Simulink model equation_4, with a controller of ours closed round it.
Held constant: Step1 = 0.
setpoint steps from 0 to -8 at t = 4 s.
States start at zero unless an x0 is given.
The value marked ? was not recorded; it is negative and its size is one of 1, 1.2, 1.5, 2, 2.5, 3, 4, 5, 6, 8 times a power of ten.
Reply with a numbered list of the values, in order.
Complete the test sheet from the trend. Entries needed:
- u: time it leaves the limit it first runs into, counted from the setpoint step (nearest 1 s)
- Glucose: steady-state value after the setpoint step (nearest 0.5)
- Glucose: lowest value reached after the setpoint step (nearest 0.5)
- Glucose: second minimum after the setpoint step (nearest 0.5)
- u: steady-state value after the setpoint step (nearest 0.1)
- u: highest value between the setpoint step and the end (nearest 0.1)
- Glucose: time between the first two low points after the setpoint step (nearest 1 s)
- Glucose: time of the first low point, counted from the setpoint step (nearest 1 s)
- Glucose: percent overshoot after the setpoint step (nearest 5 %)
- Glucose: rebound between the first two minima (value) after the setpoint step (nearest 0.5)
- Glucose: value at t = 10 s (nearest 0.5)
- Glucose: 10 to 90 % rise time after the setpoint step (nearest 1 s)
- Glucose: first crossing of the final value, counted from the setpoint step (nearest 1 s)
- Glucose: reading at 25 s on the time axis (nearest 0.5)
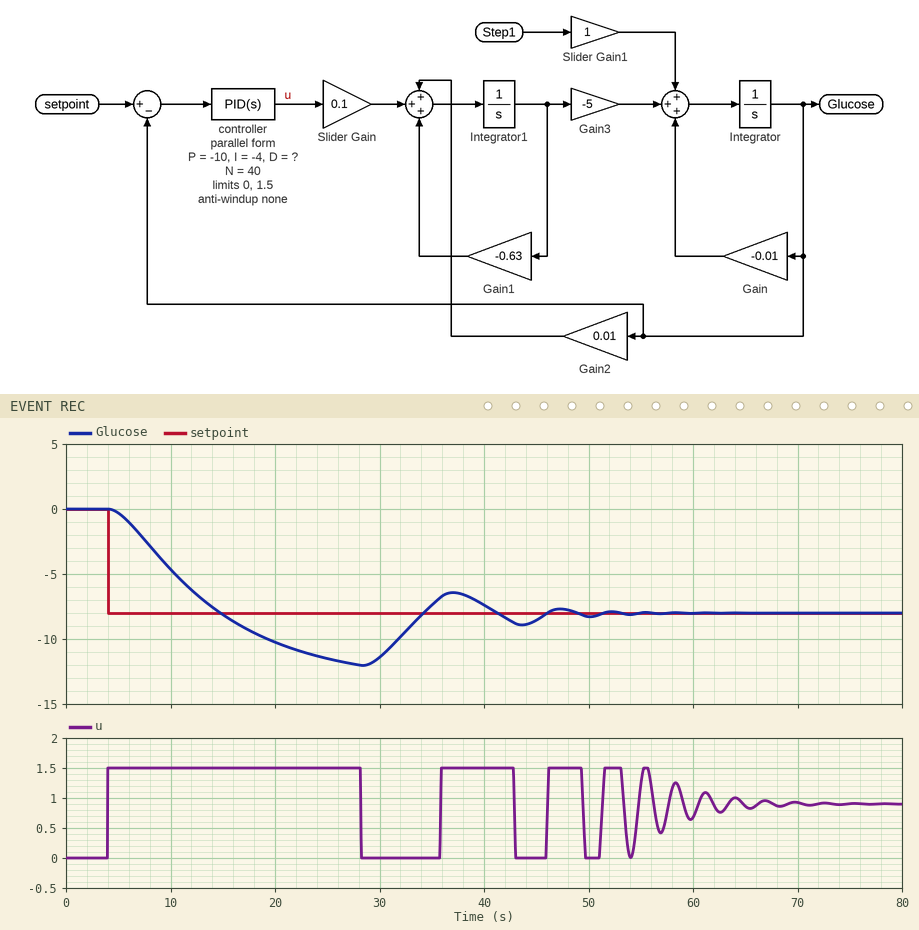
1. 24 s
2. -8.0
3. -12.0
4. -9.0
5. 0.9
6. 1.5
7. 15 s
8. 24 s
9. 50 %
10. -6.5
11. -4.5
12. 8 s
13. 11 s
14. -11.5
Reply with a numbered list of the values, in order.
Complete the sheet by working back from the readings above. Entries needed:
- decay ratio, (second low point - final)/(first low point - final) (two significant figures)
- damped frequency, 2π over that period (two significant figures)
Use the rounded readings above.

1. 0.25
2. 0.42 rad/s
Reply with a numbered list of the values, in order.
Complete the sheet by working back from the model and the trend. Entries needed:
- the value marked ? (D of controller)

1. -0.4
